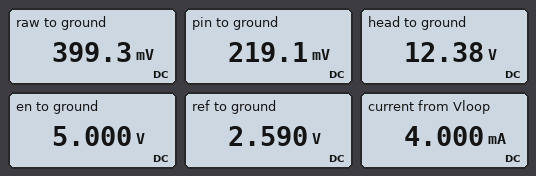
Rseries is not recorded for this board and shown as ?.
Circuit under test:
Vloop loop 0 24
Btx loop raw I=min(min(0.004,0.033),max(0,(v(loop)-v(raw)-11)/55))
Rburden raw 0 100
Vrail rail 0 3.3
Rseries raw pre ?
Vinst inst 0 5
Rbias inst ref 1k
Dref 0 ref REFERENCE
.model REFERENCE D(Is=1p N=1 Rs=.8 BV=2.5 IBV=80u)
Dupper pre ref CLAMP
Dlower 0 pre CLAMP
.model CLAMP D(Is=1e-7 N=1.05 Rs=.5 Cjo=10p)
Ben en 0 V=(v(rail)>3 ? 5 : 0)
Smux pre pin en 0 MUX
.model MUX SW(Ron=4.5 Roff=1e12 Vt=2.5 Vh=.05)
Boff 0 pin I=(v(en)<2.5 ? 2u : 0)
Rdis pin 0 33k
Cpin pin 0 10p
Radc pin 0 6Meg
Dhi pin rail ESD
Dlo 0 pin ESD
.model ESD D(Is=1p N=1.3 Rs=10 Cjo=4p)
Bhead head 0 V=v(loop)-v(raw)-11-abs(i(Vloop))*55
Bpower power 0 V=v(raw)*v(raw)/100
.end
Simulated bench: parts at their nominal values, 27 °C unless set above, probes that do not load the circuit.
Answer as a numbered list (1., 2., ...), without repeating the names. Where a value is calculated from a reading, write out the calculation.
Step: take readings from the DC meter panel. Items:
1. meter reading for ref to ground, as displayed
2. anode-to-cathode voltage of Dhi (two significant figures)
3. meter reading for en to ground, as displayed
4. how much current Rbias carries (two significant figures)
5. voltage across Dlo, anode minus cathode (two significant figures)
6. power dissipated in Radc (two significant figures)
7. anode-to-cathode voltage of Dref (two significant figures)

1. 2.590 V
2. 219.1 mV - 3.3 V = -3.1 V
3. 5.000 V
4. (5 V - 2.59 V) / 1 kΩ = 2.4 mA
5. 0 V - 219.1 mV = -220 mV
6. (219.1 mV)^2 / 6 MΩ = 8.0 nW
7. 0 V - 2.59 V = -2.6 V
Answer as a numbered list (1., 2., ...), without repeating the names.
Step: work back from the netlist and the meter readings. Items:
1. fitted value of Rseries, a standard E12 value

1. 27 kΩ
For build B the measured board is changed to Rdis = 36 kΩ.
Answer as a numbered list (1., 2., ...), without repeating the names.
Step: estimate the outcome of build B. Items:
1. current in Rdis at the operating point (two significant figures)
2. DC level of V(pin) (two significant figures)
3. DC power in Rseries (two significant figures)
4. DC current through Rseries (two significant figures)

1. 6.3 µA
2. 230 mV
3. 1.1 µW
4. 6.4 µA
